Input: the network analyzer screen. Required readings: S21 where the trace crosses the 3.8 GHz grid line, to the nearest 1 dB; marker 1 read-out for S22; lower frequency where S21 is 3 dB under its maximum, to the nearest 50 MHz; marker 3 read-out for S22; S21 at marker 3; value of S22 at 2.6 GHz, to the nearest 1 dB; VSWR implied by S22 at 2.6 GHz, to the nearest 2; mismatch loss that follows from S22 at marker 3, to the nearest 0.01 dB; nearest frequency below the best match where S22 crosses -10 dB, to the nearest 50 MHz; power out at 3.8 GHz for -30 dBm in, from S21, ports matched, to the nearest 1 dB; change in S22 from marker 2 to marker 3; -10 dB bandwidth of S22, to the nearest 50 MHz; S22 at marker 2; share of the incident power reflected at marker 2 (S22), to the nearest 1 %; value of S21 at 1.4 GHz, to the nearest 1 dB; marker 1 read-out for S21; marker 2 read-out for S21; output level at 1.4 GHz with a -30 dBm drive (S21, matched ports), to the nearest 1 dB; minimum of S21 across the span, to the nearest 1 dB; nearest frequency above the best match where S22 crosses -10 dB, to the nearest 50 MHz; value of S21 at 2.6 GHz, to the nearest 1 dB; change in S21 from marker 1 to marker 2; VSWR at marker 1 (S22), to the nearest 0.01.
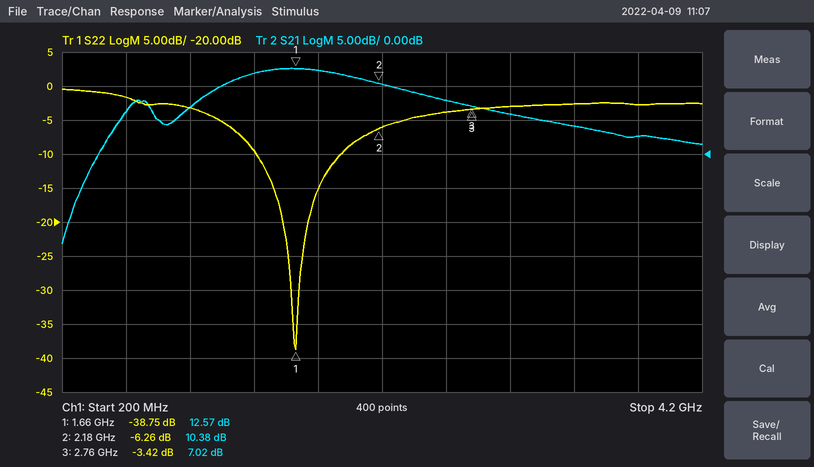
3 dB
-38.75 dB
1.15 GHz
-3.42 dB
7.02 dB
-4 dB
4
2.64 dB
1.40 GHz
-27 dBm
2.84 dB
550 MHz
-6.26 dB
24 %
12 dB
12.57 dB
10.38 dB
-18 dBm
-13 dB
1.95 GHz
8 dB
-2.19 dB
1.02
